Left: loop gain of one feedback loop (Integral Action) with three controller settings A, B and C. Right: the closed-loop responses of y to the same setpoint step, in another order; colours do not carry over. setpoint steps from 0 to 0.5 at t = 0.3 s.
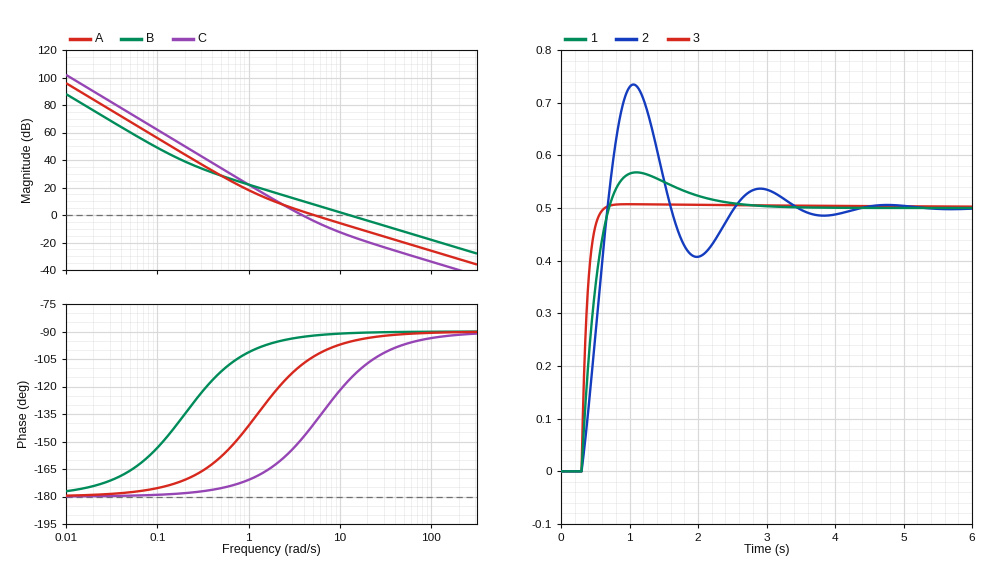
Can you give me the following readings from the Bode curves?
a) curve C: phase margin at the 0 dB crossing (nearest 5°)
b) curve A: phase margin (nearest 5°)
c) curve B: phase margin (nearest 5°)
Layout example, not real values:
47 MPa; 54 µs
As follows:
30°; 75°; 90°
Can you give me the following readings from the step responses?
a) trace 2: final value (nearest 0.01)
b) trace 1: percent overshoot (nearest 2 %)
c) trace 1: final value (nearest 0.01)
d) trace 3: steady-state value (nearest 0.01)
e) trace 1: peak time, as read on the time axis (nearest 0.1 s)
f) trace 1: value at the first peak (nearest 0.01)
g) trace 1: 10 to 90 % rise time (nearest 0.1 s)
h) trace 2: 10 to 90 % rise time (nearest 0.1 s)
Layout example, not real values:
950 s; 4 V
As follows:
0.50; 14 %; 0.50; 0.50; 1.1 s; 0.57; 0.3 s; 0.3 s
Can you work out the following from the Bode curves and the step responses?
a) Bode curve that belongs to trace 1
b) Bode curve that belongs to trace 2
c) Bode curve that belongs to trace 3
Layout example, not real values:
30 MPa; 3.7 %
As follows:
A; C; B
